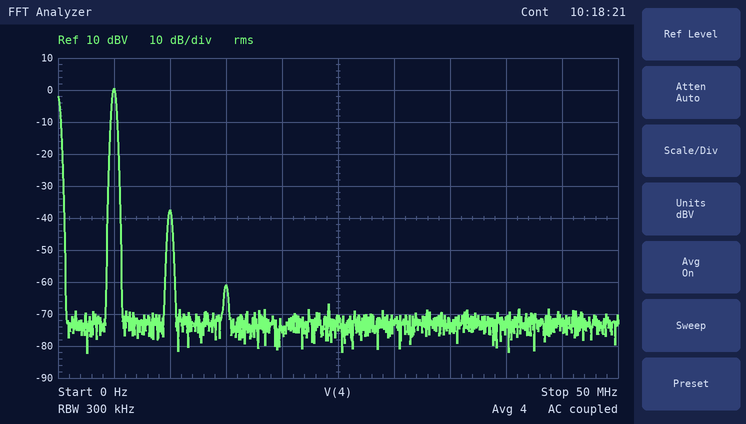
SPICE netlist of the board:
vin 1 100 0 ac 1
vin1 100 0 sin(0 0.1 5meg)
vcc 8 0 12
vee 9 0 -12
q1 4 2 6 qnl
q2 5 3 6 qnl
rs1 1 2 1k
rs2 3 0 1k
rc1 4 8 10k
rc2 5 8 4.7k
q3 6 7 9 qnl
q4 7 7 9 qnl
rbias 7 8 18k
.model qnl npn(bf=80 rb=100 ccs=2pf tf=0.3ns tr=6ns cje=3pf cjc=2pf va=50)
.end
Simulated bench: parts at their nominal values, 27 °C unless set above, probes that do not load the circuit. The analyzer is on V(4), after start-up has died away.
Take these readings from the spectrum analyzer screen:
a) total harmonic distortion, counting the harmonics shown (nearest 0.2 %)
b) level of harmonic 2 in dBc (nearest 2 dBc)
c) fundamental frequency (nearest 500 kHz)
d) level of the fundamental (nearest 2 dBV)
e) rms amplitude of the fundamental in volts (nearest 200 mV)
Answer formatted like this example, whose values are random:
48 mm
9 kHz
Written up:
1.2 %
-38 dBc
5.0 MHz
0 dBV
1.0 V
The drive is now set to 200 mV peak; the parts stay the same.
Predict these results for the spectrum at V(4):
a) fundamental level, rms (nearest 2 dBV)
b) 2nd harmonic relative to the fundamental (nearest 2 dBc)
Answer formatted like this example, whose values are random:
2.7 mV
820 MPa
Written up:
6 dBV
-32 dBc
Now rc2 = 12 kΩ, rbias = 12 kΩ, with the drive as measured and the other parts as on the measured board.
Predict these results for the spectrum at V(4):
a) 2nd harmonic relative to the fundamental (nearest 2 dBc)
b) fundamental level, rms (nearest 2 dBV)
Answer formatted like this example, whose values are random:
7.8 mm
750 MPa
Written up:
-22 dBc
-8 dBV
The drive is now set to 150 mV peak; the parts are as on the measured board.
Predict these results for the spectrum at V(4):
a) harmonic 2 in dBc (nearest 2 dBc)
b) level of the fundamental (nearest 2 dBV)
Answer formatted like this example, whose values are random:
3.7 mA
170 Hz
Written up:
-34 dBc
4 dBV
